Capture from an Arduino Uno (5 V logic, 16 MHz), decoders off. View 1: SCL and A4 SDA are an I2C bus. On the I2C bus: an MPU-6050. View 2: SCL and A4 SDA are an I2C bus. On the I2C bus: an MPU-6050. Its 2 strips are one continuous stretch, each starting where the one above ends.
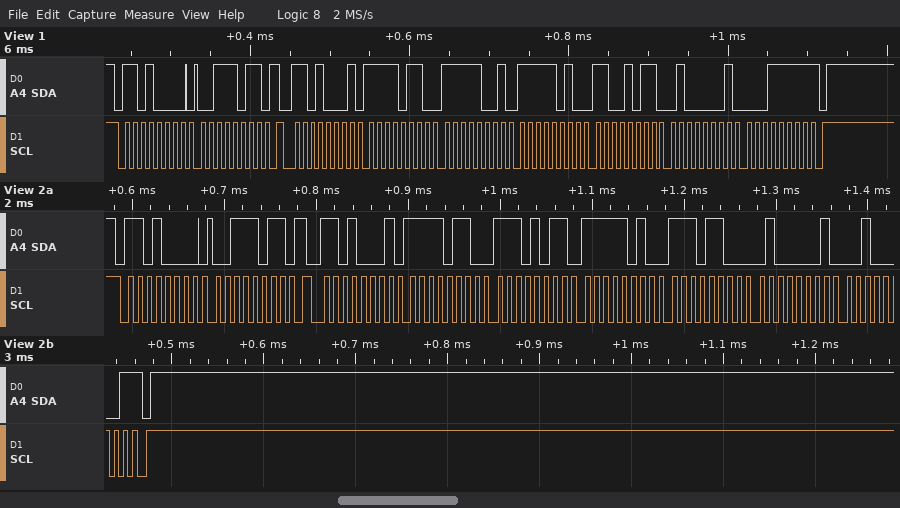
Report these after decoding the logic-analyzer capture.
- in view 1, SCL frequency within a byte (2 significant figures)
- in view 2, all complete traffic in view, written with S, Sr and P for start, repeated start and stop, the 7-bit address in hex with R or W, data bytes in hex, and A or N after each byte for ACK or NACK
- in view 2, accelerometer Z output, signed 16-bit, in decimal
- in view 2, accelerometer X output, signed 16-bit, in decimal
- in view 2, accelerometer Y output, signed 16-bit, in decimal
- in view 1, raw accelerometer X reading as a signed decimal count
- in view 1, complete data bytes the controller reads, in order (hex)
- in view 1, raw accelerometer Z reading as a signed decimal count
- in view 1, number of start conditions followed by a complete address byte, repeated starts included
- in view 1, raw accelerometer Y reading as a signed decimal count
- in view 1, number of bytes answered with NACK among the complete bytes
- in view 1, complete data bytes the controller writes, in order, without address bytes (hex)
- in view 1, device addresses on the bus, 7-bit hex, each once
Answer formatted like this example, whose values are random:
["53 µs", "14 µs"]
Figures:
["100 kHz", "S 68W A 3B A Sr 68R A F6 A EB A FA A EC A 41 A 21 N P", "16673", "-2325", "-1300", "-2311", "F6 F9 FA CB 41 1F", "16671", "2", "-1333", "1", "3B", "0x68"]
